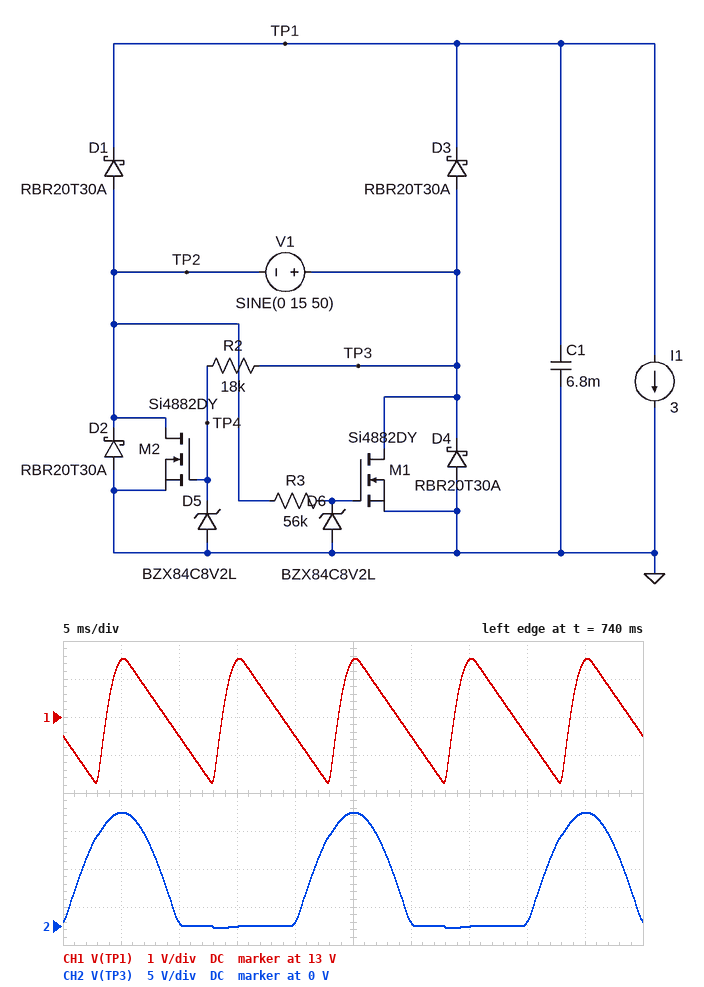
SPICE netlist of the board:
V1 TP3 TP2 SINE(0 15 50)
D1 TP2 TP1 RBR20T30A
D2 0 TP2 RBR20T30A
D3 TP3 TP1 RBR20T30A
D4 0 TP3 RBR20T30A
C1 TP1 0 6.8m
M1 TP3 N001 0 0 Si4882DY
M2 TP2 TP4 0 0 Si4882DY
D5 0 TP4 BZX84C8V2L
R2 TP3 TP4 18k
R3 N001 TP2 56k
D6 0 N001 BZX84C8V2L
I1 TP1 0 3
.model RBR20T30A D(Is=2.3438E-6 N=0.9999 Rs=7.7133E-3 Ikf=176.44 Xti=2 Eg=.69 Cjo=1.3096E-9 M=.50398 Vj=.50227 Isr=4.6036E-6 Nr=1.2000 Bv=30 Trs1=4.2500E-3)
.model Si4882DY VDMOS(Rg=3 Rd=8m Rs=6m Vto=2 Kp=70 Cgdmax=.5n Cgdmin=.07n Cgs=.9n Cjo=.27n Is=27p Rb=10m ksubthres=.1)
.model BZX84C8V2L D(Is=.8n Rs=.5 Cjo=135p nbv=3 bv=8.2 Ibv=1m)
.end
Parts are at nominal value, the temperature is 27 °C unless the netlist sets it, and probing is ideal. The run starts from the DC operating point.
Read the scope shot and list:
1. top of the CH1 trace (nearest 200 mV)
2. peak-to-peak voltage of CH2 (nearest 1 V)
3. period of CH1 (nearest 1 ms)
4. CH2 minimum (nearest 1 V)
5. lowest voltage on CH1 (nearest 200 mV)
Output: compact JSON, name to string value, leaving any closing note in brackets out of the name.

{"top of the CH1 trace": "14.6 V", "peak-to-peak voltage of CH2": "15 V", "period of CH1": "10 ms", "CH2 minimum": "0 V", "lowest voltage on CH1": "11.2 V"}
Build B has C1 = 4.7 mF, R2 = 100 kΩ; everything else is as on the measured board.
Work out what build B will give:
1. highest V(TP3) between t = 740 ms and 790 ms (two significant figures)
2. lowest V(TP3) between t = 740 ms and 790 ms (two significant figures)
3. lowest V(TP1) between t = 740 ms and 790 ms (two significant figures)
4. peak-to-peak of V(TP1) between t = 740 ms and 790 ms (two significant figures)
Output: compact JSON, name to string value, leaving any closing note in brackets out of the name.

{"highest V(TP3) between t = 740 ms and 790 ms": "15 V", "lowest V(TP3) between t = 740 ms and 790 ms": "-270 mV", "lowest V(TP1) between t = 740 ms and 790 ms": "10 V", "peak-to-peak of V(TP1) between t = 740 ms and 790 ms": "4.5 V"}
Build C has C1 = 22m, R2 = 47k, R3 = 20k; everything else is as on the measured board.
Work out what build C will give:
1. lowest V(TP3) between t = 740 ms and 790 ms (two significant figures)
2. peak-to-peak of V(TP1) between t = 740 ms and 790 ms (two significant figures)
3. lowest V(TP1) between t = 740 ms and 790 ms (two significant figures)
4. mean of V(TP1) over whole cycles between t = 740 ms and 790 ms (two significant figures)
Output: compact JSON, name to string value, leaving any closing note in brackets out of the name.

{"lowest V(TP3) between t = 740 ms and 790 ms": "-360 mV", "peak-to-peak of V(TP1) between t = 740 ms and 790 ms": "1.1 V", "lowest V(TP1) between t = 740 ms and 790 ms": "13 V", "mean of V(TP1) over whole cycles between t = 740 ms and 790 ms": "14 V"}
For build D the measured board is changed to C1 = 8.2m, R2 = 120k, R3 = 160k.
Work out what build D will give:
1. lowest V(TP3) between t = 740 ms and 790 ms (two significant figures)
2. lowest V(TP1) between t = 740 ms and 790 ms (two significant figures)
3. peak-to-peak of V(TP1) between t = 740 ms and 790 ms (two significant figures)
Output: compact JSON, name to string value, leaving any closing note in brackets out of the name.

{"lowest V(TP3) between t = 740 ms and 790 ms": "-320 mV", "lowest V(TP1) between t = 740 ms and 790 ms": "12 V", "peak-to-peak of V(TP1) between t = 740 ms and 790 ms": "2.8 V"}
